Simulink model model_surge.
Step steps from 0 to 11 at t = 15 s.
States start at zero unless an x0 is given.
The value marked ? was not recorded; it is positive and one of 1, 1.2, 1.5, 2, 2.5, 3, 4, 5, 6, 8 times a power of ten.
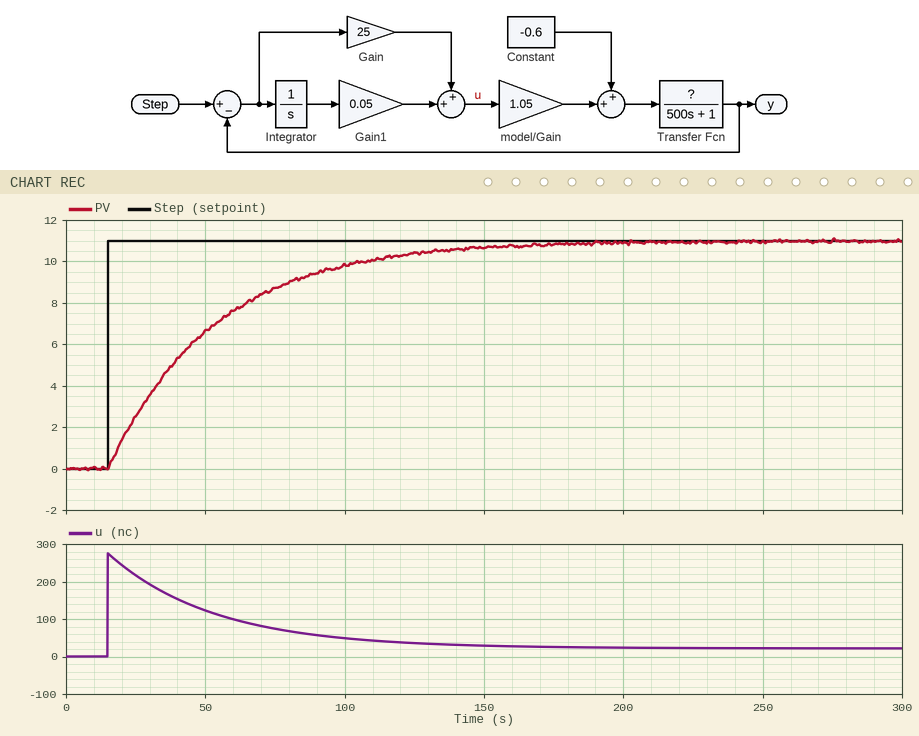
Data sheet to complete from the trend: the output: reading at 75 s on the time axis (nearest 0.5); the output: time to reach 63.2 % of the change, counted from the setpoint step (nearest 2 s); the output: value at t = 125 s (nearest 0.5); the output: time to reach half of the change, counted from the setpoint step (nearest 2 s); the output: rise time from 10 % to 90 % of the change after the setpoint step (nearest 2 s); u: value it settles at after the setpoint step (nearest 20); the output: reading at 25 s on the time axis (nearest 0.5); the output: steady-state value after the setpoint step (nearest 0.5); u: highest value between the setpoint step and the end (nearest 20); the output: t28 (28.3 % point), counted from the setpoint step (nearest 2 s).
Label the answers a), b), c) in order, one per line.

a) 8.5
b) 38 s
c) 10.5
d) 26 s
e) 84 s
f) 20
g) 2.5
h) 11.0
i) 280
j) 12 s
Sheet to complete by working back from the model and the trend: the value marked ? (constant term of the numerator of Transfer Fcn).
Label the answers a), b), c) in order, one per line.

a) 0.5
